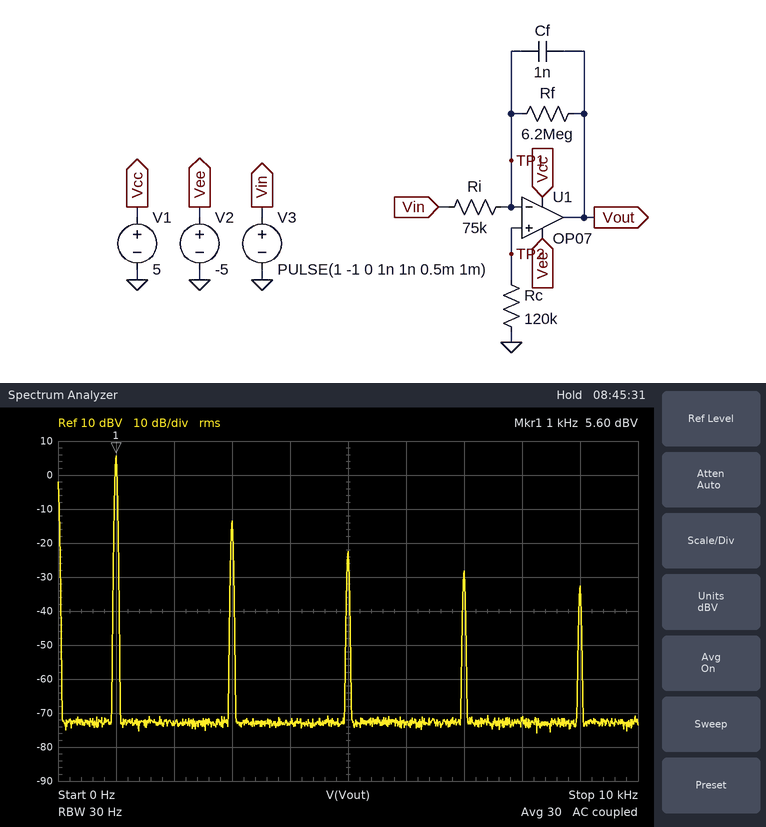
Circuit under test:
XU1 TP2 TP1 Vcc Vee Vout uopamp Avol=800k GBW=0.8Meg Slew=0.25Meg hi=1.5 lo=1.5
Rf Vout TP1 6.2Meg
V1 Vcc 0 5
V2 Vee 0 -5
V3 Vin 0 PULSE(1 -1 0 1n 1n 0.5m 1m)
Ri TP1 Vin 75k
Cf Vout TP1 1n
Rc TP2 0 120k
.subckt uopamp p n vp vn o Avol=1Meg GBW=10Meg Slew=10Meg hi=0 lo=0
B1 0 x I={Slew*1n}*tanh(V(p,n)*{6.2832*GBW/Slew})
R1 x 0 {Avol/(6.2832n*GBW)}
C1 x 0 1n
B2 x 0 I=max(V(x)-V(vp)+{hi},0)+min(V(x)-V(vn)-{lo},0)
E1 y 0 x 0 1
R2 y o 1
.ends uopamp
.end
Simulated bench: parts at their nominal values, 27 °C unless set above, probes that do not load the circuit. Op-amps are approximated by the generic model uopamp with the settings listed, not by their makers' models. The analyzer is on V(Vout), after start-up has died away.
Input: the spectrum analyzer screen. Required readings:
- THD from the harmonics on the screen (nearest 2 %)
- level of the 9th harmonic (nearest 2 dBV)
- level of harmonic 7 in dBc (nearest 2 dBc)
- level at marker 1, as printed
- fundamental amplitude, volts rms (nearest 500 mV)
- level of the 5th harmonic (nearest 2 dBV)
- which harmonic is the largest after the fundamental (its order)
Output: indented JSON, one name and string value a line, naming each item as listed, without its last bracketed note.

{
  "THD from the harmonics on the screen": "12 %",
  "level of the 9th harmonic": "-32 dBV",
  "level of harmonic 7 in dBc": "-34 dBc",
  "level at marker 1, as printed": "5.60 dBV",
  "fundamental amplitude, volts rms": "2.0 V",
  "level of the 5th harmonic": "-22 dBV",
  "which harmonic is the largest after the fundamental": "3"
}
